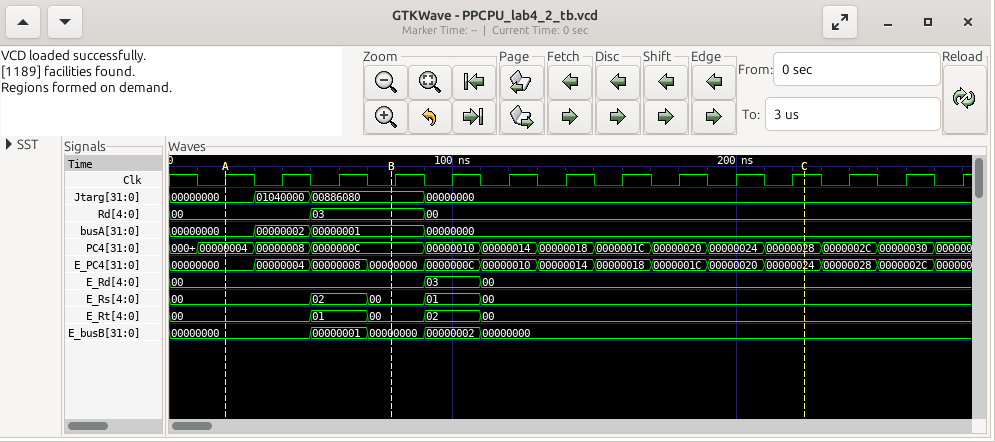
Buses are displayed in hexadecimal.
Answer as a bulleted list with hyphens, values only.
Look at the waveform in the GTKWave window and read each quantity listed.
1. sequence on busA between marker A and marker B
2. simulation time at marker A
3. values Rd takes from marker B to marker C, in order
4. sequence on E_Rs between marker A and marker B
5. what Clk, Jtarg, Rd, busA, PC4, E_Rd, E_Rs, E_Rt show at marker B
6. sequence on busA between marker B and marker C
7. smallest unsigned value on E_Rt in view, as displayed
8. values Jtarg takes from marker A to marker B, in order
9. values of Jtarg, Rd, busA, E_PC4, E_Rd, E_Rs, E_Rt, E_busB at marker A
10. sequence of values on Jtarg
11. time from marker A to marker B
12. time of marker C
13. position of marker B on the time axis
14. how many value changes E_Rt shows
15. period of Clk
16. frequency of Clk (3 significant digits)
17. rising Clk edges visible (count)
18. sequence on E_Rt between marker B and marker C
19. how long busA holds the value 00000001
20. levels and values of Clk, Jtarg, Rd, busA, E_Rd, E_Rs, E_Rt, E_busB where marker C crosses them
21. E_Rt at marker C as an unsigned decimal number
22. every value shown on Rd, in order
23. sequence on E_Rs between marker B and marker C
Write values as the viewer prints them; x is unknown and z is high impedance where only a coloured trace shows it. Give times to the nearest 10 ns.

- 00000000, 00000002, 00000001
- 20 ns
- 03, 00
- 00, 02, 00
- Clk=0, Jtarg=00886080, Rd=03, busA=00000001, PC4=0000000C, E_Rd=00, E_Rs=00, E_Rt=00
- 00000001, 00000000
- 00
- 00000000, 01040000, 00886080
- Jtarg=00000000, Rd=00, busA=00000000, E_PC4=00000000, E_Rd=00, E_Rs=00, E_Rt=00, E_busB=00000000
- 00000000, 01040000, 00886080, 00000000
- 60 ns
- 220 ns
- 80 ns
- 4
- 20 ns
- 50.0 MHz
- 14
- 00, 02, 00
- 40 ns
- Clk=1, Jtarg=00000000, Rd=00, busA=00000000, E_Rd=00, E_Rs=00, E_Rt=00, E_busB=00000000
- 0
- 00, 03, 00
- 00, 01, 00
